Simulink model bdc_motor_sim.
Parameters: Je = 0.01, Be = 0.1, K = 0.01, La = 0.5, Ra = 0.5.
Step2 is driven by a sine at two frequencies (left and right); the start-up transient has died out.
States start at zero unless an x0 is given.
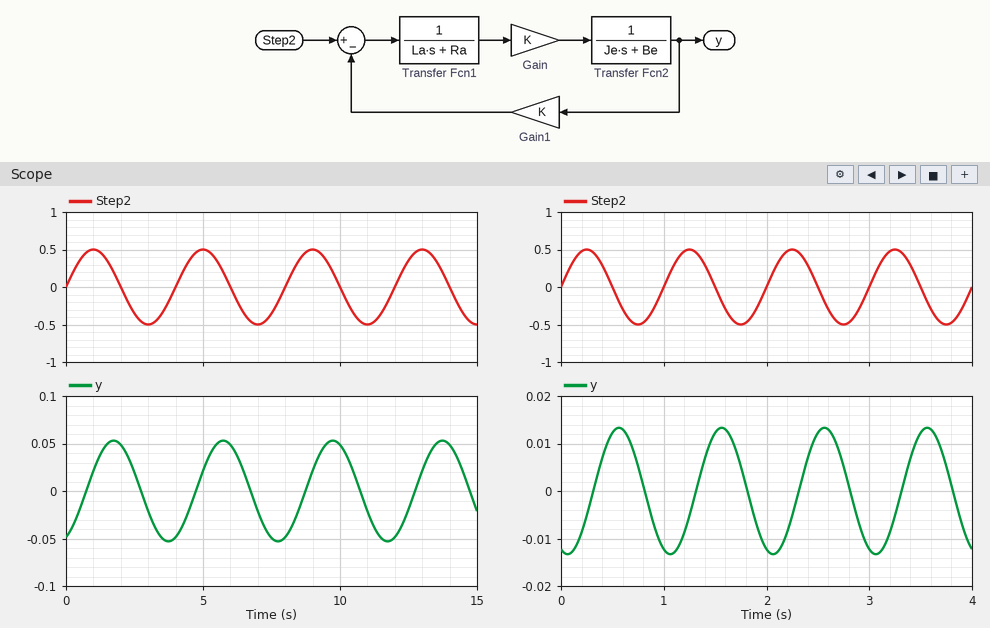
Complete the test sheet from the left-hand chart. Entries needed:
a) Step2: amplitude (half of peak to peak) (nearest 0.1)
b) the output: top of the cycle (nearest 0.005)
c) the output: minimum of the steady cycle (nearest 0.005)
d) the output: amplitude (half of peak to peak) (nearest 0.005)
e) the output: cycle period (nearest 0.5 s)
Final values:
0.5
0.055
-0.055
0.055
4.0 s
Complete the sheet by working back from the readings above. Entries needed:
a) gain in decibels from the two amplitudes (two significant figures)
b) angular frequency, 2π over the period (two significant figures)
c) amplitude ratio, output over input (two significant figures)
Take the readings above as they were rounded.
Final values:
-19 dB
1.6 rad/s
0.11
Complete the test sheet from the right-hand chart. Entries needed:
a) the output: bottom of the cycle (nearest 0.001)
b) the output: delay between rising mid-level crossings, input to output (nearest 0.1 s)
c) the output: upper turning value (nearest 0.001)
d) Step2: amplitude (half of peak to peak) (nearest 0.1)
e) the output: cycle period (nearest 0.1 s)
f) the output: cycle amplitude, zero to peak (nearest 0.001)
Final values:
-0.013
0.3 s
0.013
0.5
1.0 s
0.013
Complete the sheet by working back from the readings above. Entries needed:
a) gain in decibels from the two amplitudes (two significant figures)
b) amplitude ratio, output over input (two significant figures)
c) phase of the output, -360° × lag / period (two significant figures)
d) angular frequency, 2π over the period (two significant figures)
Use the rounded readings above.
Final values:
-32 dB
0.026
-110°
6.3 rad/s
